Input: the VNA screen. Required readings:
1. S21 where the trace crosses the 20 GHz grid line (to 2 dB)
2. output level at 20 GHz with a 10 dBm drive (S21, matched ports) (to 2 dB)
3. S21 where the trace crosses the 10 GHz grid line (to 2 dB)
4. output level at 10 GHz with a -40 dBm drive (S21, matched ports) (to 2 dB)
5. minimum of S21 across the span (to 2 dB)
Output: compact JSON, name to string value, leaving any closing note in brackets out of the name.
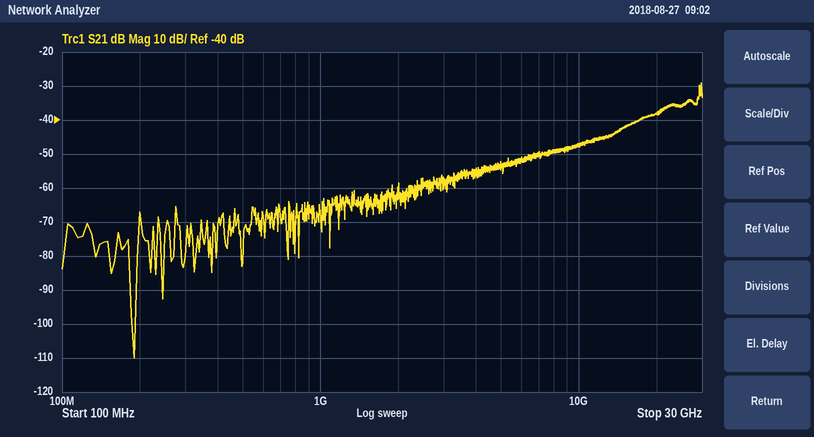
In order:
{"S21 where the trace crosses the 20 GHz grid line": "-38 dB", "output level at 20 GHz with a 10 dBm drive (S21, matched ports)": "-28 dBm", "S21 where the trace crosses the 10 GHz grid line": "-48 dB", "output level at 10 GHz with a -40 dBm drive (S21, matched ports)": "-88 dBm", "minimum of S21 across the span": "-110 dB"}
